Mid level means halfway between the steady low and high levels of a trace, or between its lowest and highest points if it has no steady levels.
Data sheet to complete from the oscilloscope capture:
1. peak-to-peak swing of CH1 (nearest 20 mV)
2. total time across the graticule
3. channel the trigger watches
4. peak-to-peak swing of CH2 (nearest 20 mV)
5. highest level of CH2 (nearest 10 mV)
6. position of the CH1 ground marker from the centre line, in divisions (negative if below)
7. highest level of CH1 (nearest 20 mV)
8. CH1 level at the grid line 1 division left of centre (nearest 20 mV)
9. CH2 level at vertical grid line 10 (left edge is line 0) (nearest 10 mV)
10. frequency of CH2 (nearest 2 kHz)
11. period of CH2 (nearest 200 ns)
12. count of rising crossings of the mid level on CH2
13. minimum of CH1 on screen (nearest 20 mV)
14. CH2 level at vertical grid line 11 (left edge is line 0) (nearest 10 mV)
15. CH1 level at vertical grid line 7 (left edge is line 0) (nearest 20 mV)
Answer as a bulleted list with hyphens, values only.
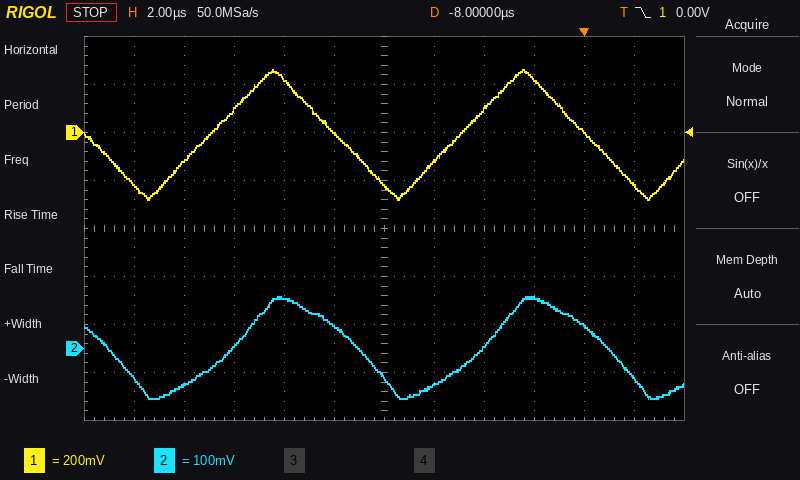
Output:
- 540 mV
- 24 µs
- CH1
- 220 mV
- 110 mV
- +2.0 div
- 260 mV
- 0 mV
- 50 mV
- 100 kHz
- 10.0 µs
- 2
- -280 mV
- -60 mV
- -120 mV
